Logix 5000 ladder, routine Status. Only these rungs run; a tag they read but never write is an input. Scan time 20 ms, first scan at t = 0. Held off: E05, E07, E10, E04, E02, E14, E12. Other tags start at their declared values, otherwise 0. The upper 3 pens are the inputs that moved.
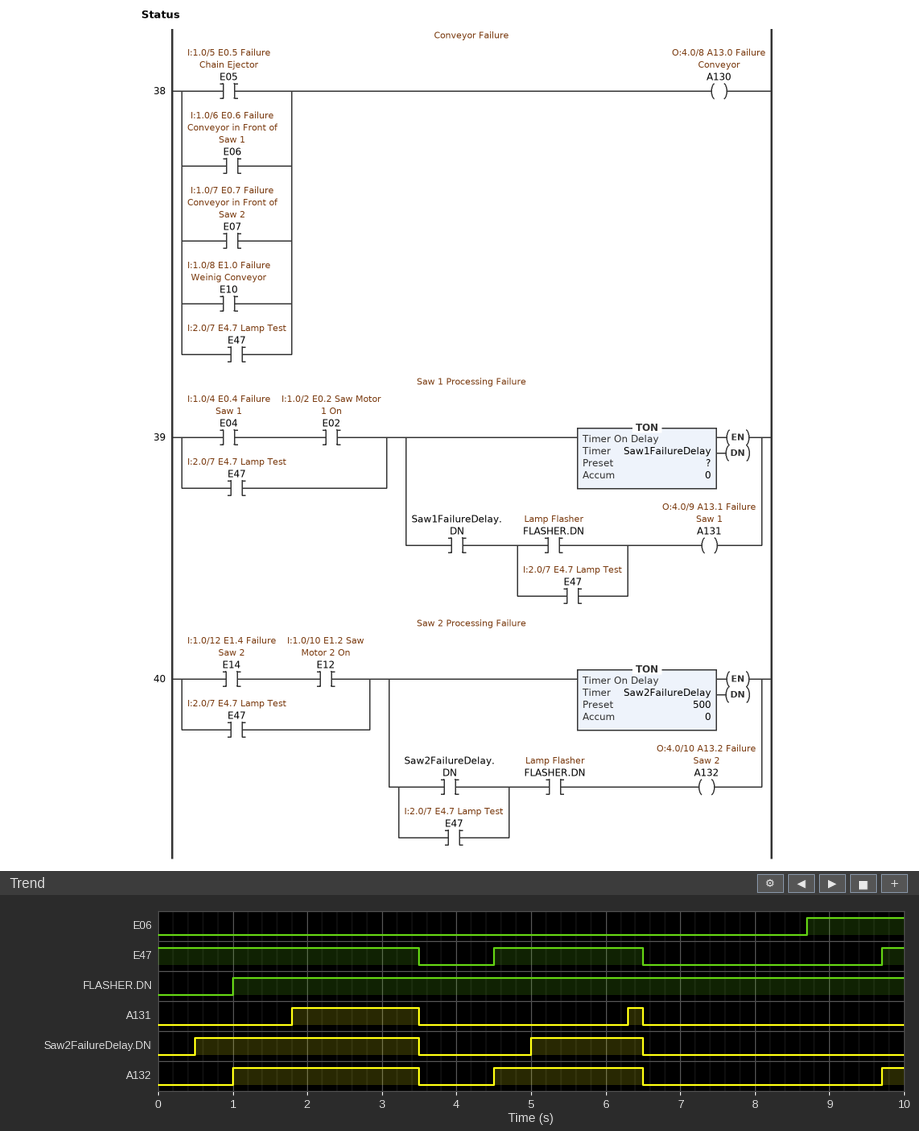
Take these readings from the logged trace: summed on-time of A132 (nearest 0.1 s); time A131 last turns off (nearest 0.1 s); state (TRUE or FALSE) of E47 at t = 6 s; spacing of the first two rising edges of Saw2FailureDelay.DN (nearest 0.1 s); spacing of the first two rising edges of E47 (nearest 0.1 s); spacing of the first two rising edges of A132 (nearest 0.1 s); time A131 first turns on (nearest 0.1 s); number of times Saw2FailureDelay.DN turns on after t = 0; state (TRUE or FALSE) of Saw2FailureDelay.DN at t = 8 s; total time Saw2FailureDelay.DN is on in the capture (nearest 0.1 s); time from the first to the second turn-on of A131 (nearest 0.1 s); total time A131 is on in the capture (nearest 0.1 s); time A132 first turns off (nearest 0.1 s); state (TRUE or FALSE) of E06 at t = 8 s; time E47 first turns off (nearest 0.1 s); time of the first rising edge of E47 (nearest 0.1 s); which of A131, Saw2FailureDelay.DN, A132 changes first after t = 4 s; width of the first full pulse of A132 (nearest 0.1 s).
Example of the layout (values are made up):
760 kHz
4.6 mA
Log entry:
4.8 s
6.5 s
TRUE
4.5 s
5.2 s
3.5 s
1.8 s
2
FALSE
4.5 s
4.5 s
1.9 s
3.5 s
FALSE
3.5 s
4.5 s
A132
2.5 s
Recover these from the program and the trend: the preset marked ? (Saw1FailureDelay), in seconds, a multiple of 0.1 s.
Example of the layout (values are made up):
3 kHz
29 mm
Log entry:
1.8 s
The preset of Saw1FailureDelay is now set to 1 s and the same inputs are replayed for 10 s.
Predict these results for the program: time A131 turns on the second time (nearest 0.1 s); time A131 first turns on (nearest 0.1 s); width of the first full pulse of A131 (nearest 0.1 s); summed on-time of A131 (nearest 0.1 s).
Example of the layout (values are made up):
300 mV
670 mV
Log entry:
5.5 s
1.0 s
2.5 s
3.5 s
